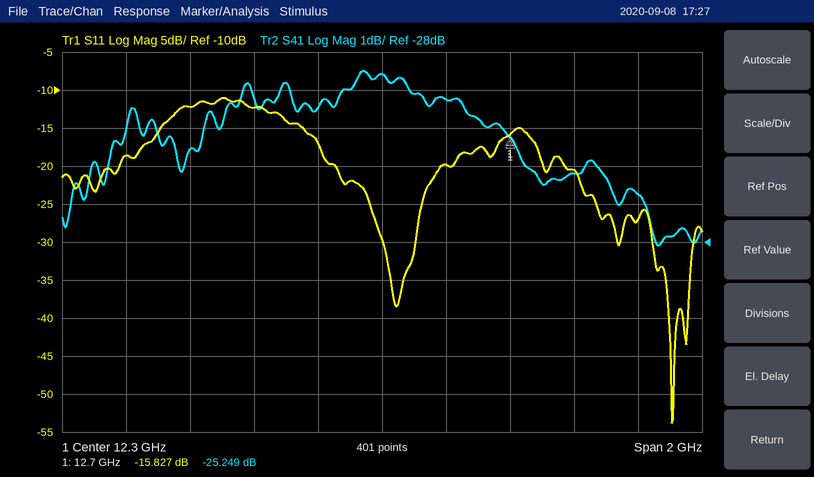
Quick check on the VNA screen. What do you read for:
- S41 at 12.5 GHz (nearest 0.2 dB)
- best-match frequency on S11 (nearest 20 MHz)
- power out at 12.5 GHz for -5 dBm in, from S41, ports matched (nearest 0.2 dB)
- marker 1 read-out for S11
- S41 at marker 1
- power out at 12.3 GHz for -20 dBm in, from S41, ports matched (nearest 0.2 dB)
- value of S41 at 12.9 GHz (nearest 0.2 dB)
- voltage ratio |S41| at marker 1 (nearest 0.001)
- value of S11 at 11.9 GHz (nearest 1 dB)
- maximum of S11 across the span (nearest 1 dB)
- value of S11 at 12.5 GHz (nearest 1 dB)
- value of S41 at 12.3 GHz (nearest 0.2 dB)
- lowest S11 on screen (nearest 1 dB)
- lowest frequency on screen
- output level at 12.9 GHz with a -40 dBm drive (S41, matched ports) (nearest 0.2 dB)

-24.2 dB
13.20 GHz
-29.2 dBm
-15.827 dB
-25.249 dB
-43.6 dBm
-26.2 dB
0.055
-12 dB
-11 dB
-20 dB
-23.6 dB
-54 dB
11.3 GHz
-66.2 dBm
